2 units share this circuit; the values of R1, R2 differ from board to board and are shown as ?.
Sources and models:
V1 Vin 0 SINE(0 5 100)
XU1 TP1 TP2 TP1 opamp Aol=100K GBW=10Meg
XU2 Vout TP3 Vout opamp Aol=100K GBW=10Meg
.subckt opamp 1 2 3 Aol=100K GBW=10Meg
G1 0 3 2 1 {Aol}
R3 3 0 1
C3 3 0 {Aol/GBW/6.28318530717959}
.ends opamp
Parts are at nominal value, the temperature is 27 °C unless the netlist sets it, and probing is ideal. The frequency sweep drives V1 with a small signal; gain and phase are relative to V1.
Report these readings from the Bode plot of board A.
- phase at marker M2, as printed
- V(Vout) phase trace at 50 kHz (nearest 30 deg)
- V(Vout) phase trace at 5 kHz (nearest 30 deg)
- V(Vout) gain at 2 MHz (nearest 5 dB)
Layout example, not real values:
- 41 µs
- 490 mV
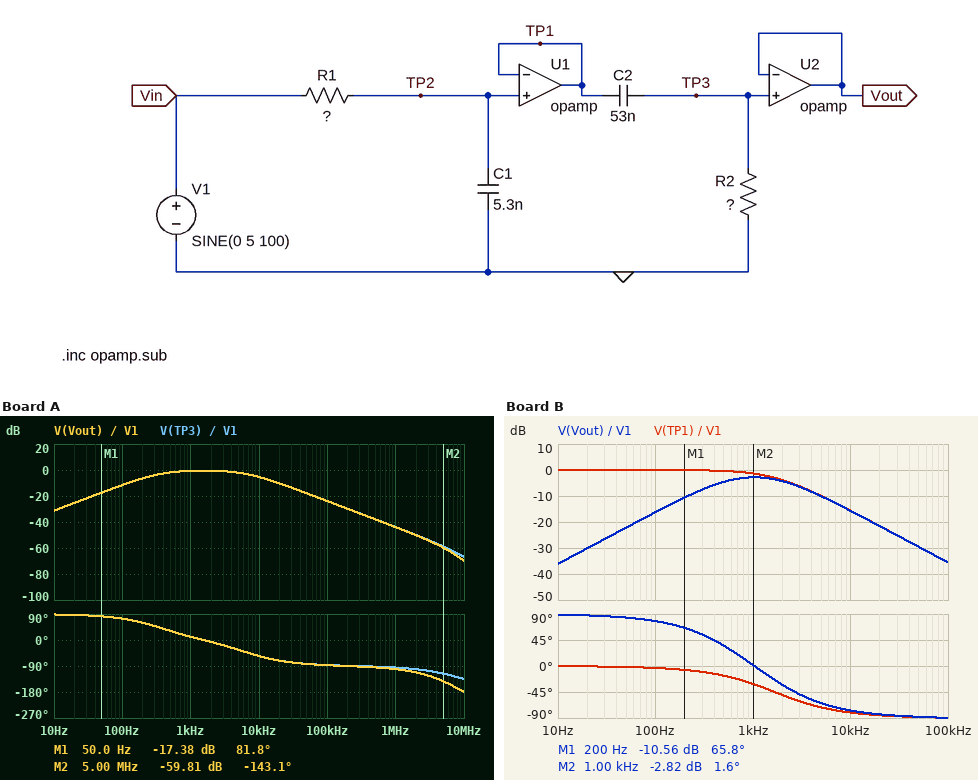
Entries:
- -143.1 deg
- -90 deg
- -30 deg
- -50 dB
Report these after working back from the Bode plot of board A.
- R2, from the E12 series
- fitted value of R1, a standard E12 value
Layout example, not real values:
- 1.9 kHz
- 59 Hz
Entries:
- 8.2 kΩ
- 4.7 kΩ
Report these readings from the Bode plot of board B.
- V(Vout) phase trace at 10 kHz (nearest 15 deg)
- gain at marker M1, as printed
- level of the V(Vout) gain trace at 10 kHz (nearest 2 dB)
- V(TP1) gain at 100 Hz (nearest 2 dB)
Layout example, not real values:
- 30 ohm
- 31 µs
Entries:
- -75 deg
- -10.56 dB
- -16 dB
- 0 dB
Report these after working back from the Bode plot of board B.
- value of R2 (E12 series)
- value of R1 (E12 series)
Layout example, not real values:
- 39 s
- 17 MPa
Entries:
- 4.7 kΩ
- 18 kΩ
